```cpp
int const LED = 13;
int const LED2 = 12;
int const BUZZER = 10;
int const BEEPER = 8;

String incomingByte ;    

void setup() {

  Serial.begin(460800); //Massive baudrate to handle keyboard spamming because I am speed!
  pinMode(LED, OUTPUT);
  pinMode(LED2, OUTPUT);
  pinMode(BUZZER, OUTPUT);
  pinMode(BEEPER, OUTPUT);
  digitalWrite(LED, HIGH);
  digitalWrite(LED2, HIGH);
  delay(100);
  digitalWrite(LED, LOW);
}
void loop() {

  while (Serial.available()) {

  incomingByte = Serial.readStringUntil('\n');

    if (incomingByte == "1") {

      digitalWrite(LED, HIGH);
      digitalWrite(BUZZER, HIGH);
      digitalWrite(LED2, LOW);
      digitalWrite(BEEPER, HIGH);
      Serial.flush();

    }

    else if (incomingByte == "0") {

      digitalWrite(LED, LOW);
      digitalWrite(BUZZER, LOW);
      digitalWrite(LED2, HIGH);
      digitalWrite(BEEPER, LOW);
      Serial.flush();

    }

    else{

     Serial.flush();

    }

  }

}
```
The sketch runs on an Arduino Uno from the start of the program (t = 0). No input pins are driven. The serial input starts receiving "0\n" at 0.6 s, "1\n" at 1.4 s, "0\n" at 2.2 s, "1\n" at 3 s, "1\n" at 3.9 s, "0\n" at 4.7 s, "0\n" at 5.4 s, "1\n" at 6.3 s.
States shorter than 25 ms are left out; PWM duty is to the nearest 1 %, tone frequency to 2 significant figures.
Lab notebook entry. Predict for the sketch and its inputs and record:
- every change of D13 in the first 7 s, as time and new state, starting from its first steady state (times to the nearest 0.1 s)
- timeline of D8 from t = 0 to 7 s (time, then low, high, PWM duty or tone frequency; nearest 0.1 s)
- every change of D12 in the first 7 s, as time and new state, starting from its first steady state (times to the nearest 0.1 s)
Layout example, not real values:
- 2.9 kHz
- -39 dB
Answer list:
- 0 s high; 0.1 s low; 1.4 s high; 2.2 s low; 3 s high; 4.7 s low; 6.3 s high
- 0 s low; 1.4 s high; 2.2 s low; 3 s high; 4.7 s low; 6.3 s high
- 0 s high; 1.4 s low; 2.2 s high; 3 s low; 4.7 s high; 6.3 s low
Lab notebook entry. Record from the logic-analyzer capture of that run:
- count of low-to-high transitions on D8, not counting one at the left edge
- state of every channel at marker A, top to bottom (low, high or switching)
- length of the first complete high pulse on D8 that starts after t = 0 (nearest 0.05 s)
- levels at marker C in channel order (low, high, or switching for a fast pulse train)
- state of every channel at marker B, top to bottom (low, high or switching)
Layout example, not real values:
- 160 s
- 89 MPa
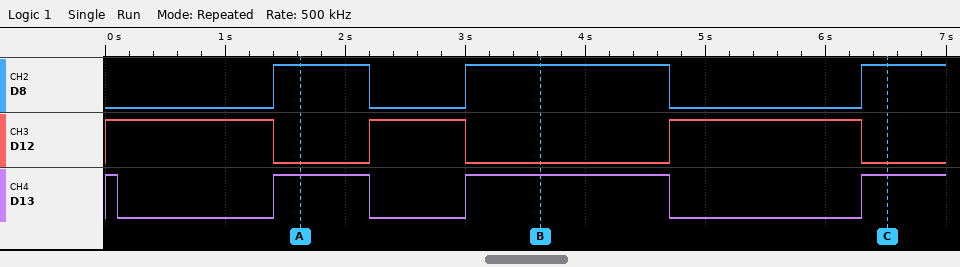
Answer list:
- 3
- D8 high, D12 low, D13 high
- 0.80 s
- D8 high, D12 low, D13 high
- D8 high, D12 low, D13 high
